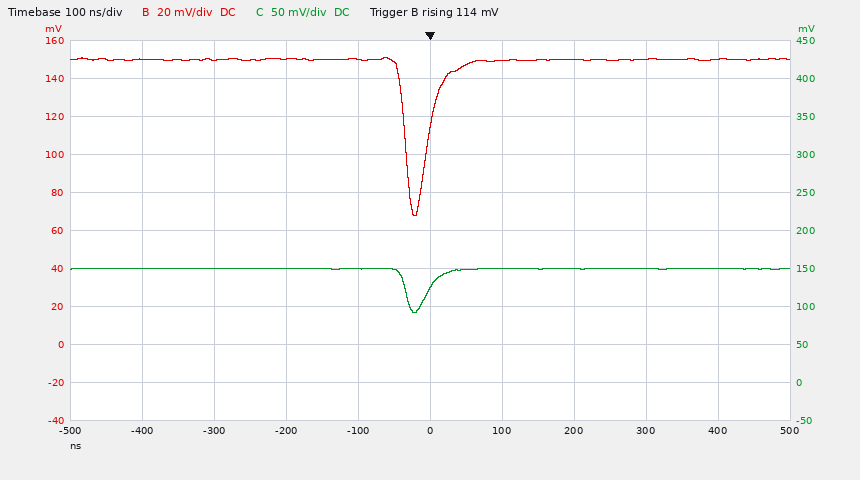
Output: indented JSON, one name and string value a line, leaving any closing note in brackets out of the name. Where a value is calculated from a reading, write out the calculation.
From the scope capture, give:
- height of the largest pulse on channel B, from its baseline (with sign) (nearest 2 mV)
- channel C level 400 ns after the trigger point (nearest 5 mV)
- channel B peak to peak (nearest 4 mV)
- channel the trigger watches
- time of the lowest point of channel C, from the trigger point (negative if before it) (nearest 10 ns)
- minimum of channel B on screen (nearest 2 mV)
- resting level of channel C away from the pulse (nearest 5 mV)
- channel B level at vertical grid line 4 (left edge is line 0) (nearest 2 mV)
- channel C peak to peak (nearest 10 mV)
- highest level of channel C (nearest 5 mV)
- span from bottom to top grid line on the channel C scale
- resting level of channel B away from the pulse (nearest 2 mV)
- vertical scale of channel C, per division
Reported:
{
  "height of the largest pulse on channel B, from its baseline (with sign)": "68 mV − (150 mV) = -82 mV",
  "channel C level 400 ns after the trigger point": "150 mV",
  "channel B peak to peak": "84 mV",
  "channel the trigger watches": "channel B",
  "time of the lowest point of channel C, from the trigger point (negative if before it)": "-20 ns",
  "minimum of channel B on screen": "68 mV",
  "resting level of channel C away from the pulse": "150 mV",
  "channel B level at vertical grid line 4 (left edge is line 0)": "150 mV",
  "channel C peak to peak": "60 mV",
  "highest level of channel C": "150 mV",
  "span from bottom to top grid line on the channel C scale": "500 mV",
  "resting level of channel B away from the pulse": "150 mV",
  "vertical scale of channel C, per division": "50 mV"
}
